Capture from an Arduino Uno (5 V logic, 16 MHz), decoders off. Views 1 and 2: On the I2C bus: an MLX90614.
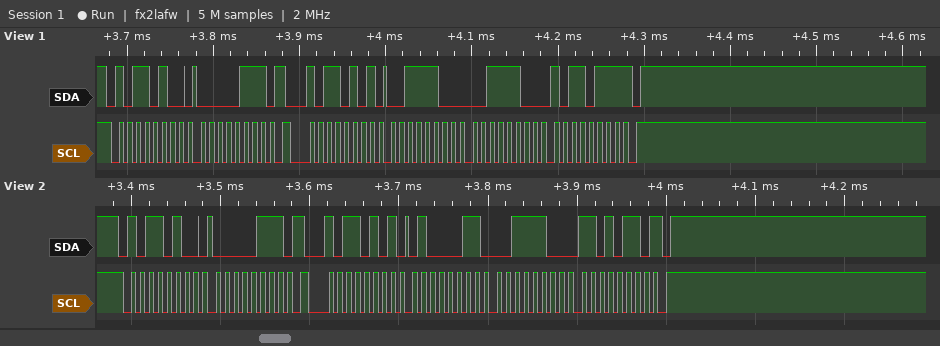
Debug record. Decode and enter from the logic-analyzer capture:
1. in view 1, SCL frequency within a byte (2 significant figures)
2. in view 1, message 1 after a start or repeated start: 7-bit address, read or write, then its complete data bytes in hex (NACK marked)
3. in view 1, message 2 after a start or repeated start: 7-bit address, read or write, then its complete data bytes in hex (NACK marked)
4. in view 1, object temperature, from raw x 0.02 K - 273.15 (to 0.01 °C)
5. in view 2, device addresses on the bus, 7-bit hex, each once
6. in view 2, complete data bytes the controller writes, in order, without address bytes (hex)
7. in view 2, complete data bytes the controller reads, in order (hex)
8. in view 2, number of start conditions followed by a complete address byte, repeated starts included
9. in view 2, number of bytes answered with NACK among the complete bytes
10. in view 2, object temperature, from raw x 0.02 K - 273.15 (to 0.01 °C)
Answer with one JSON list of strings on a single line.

["100 kHz", "0x5A write: 07", "0x5A read: 3C 3C B7 NACK", "35.25 °C", "0x5A", "07", "43 3C D6", "2", "1", "35.39 °C"]
